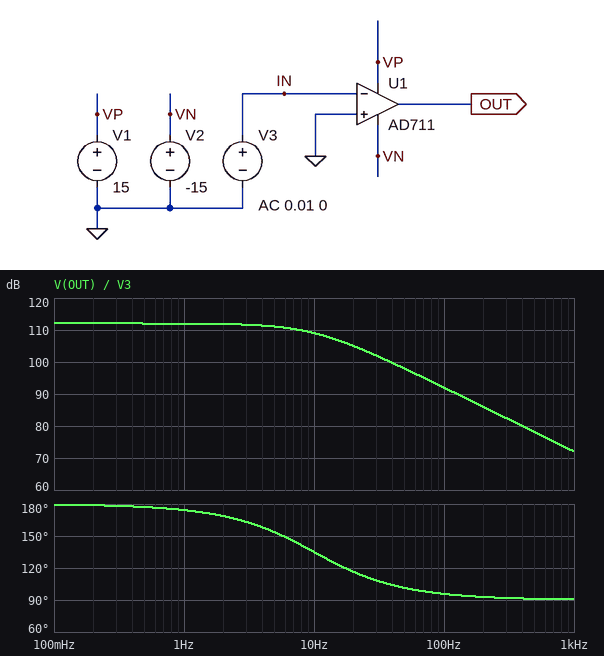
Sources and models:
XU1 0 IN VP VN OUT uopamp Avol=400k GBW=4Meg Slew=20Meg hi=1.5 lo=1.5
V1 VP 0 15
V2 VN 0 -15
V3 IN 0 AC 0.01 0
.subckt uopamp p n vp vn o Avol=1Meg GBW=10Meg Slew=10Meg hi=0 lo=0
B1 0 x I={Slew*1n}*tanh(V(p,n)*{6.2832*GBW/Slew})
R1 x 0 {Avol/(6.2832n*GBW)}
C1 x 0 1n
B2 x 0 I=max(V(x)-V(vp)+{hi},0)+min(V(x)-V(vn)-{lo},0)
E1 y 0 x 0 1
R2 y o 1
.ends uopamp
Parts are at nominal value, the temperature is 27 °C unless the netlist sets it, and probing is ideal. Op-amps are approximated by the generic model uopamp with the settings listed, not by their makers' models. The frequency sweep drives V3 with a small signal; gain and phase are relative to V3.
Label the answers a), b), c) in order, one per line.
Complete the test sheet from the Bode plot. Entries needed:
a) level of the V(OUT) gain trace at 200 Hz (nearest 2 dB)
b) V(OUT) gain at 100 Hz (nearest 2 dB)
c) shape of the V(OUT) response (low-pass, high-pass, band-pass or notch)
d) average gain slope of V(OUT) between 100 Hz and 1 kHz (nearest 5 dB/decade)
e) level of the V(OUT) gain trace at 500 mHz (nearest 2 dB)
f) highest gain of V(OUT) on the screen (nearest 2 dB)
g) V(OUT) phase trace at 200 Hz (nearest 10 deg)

a) 86 dB
b) 92 dB
c) low-pass
d) -20 dB/decade
e) 112 dB
f) 112 dB
g) 90 deg
